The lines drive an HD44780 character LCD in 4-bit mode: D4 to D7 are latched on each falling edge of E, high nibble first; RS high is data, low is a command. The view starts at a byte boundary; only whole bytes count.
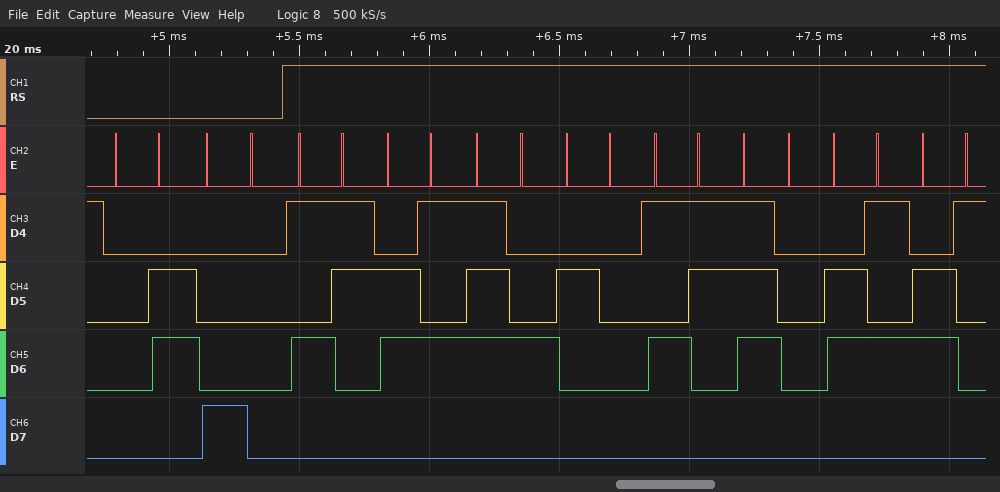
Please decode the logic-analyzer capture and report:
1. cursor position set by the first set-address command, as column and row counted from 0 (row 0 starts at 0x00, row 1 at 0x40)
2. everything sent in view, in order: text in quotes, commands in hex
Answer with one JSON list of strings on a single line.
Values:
["column 0, row 0", "0x06 0x80 \"Set Spea\""]
